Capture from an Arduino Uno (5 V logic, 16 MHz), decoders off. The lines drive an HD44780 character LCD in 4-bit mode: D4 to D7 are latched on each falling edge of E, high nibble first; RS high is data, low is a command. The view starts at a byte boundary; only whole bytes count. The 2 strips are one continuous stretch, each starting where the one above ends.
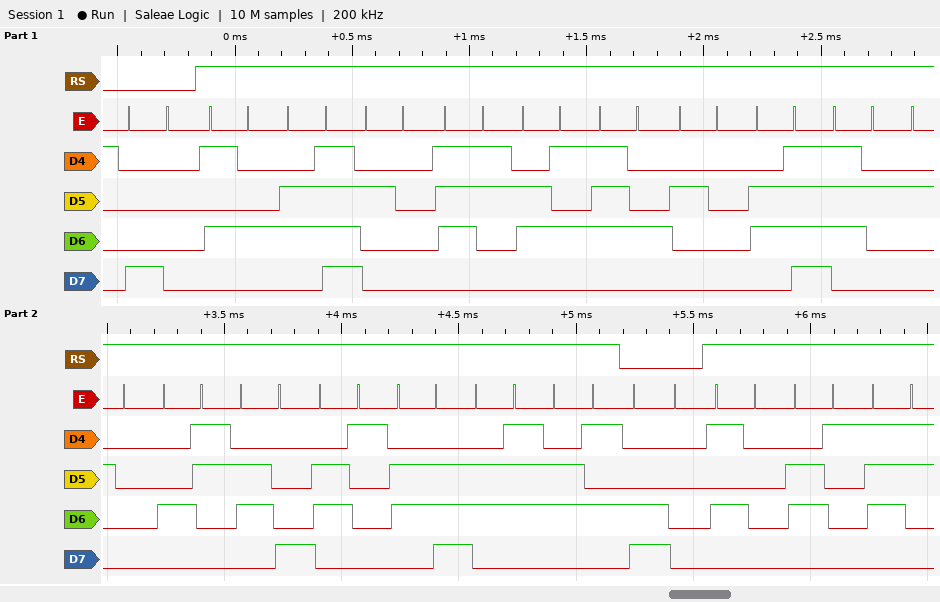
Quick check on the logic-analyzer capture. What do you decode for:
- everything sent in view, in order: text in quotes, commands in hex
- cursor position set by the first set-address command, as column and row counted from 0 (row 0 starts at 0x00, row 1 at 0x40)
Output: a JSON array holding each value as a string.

["0x80 \"To set or Change\" 0xC0 \"Pas\"", "column 0, row 0"]
